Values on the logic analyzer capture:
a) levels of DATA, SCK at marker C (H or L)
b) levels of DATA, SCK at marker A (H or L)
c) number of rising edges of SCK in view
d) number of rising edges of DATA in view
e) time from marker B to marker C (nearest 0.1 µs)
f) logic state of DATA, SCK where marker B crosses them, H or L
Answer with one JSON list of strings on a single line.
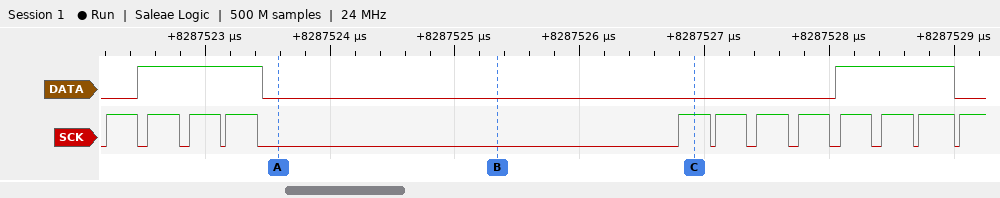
["DATA=L, SCK=H", "DATA=L, SCK=L", "12", "2", "1.6 µs", "DATA=L, SCK=L"]
